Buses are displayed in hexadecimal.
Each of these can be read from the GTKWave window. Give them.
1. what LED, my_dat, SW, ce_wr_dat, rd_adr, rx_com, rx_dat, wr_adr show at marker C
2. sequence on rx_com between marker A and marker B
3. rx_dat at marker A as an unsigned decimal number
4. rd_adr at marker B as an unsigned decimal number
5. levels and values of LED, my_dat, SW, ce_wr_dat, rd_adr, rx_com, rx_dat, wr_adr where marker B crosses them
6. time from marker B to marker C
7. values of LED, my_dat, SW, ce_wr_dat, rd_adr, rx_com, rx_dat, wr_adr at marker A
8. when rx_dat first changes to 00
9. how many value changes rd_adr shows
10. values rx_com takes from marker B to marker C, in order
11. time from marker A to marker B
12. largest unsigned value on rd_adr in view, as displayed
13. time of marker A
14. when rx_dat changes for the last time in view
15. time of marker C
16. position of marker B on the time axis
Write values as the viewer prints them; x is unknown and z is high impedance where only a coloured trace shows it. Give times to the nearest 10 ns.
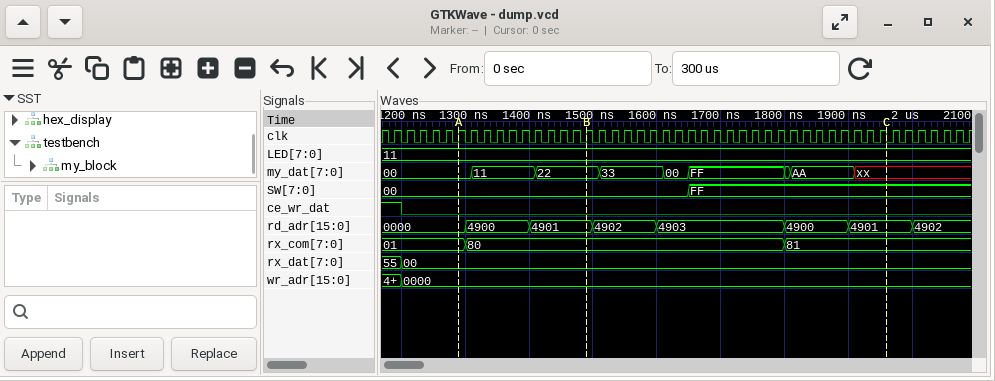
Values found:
LED=11, my_dat=xx, SW=FF, ce_wr_dat=0, rd_adr=4901, rx_com=81, rx_dat=00, wr_adr=0000
01, 80
0
18689
LED=11, my_dat=22, SW=00, ce_wr_dat=0, rd_adr=4901, rx_com=80, rx_dat=00, wr_adr=0000
470 ns
LED=11, my_dat=00, SW=00, ce_wr_dat=0, rd_adr=0000, rx_com=01, rx_dat=00, wr_adr=0000
1200 ns
7
80, 81
200 ns
4903
1290 ns
1200 ns
1960 ns
1490 ns
